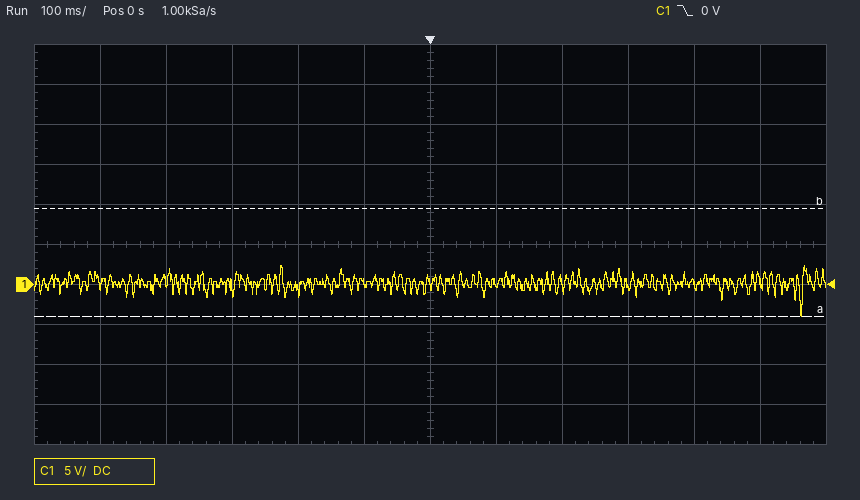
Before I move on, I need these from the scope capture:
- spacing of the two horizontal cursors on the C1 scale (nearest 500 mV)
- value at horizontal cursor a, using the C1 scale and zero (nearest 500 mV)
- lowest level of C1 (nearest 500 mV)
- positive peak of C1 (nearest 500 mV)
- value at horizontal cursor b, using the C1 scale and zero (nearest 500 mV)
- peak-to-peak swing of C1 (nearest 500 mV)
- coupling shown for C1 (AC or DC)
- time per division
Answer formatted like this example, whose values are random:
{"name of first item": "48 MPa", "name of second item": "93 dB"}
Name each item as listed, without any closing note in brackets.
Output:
{"spacing of the two horizontal cursors on the C1 scale": "13.5 V", "value at horizontal cursor a, using the C1 scale and zero": "-4.0 V", "lowest level of C1": "-4.0 V", "positive peak of C1": "2.5 V", "value at horizontal cursor b, using the C1 scale and zero": "9.5 V", "peak-to-peak swing of C1": "6.5 V", "coupling shown for C1": "DC", "time per division": "100 ms"}
